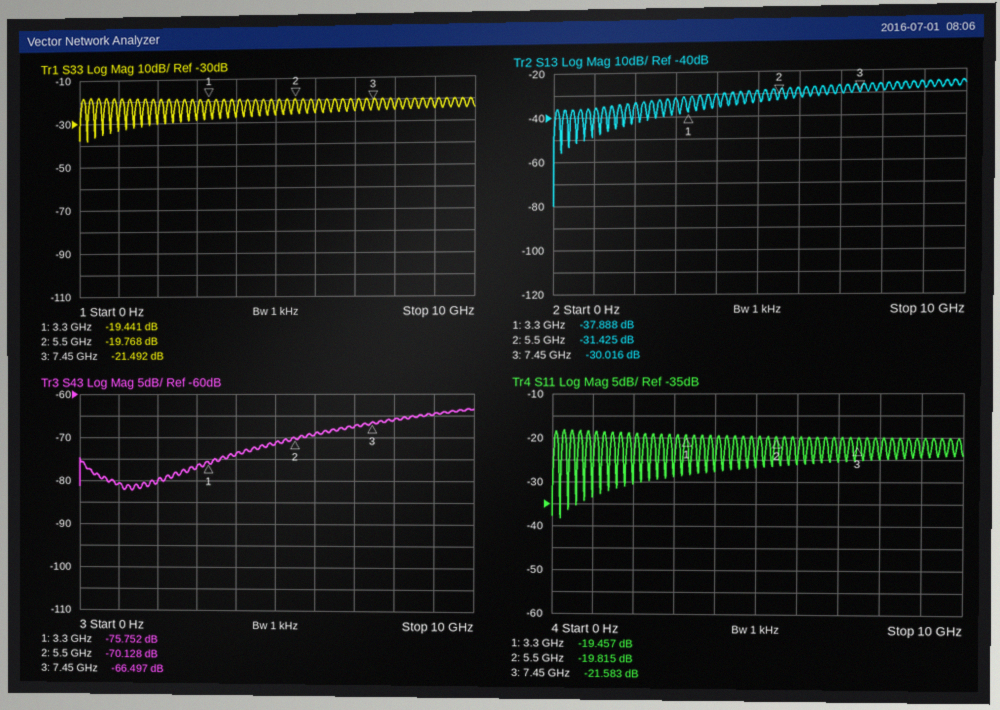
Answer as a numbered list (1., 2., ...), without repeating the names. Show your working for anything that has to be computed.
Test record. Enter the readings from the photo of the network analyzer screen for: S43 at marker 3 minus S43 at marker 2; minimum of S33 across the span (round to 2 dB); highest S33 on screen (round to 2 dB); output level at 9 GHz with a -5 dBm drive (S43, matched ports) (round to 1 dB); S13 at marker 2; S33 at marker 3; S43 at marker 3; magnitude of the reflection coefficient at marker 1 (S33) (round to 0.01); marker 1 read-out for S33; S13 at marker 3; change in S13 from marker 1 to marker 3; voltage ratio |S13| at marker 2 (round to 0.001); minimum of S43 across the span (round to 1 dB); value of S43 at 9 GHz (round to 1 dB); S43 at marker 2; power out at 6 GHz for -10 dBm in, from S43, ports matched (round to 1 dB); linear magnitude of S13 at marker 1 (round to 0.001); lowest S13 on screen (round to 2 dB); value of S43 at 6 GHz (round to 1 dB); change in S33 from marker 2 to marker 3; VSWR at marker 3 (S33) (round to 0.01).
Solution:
1. -66.497 − (-70.128) = 3.631 dB
2. -38 dB
3. -18 dB
4. -5 dBm + (-65 dB) = -70 dBm
5. -31.425 dB
6. -21.492 dB
7. -66.497 dB
8. 10^(-19.441/20) ≈ 0.11
9. -19.441 dB
10. -30.016 dB
11. -30.016 − (-37.888) = 7.872 dB
12. 10^(-31.425/20) ≈ 0.027
13. -82 dB
14. -65 dB
15. -70.128 dB
16. -10 dBm + (-69 dB) = -79 dBm
17. 10^(-37.888/20) ≈ 0.013
18. -80 dB
19. -69 dB
20. -21.492 − (-19.768) = -1.724 dB
21. (1 + 0.0842)/(1 − 0.0842) ≈ 1.18
